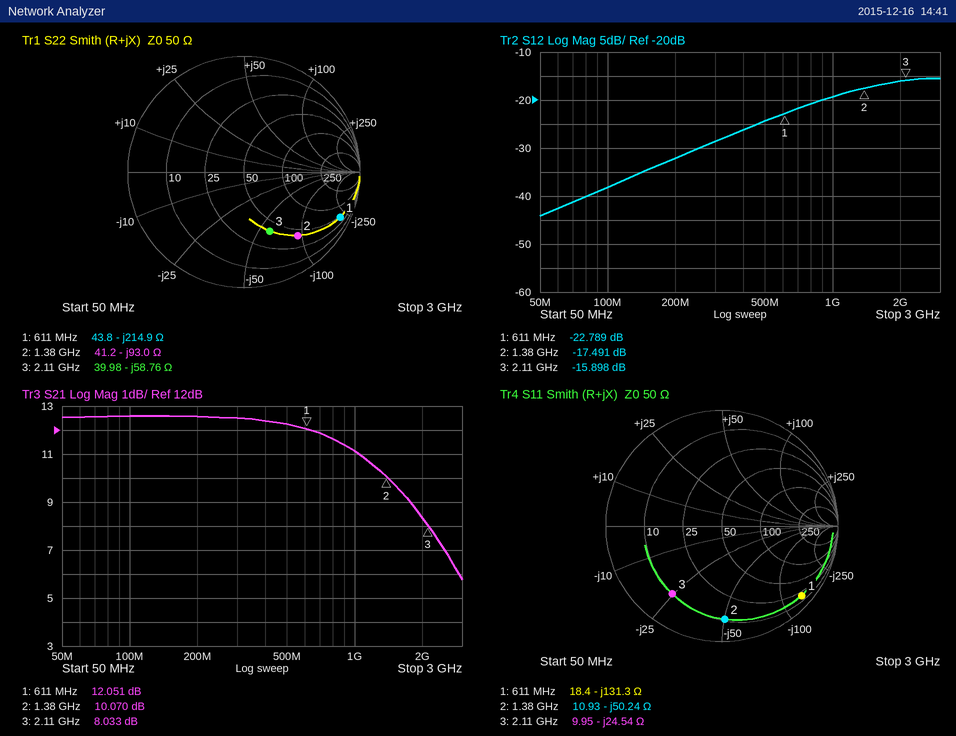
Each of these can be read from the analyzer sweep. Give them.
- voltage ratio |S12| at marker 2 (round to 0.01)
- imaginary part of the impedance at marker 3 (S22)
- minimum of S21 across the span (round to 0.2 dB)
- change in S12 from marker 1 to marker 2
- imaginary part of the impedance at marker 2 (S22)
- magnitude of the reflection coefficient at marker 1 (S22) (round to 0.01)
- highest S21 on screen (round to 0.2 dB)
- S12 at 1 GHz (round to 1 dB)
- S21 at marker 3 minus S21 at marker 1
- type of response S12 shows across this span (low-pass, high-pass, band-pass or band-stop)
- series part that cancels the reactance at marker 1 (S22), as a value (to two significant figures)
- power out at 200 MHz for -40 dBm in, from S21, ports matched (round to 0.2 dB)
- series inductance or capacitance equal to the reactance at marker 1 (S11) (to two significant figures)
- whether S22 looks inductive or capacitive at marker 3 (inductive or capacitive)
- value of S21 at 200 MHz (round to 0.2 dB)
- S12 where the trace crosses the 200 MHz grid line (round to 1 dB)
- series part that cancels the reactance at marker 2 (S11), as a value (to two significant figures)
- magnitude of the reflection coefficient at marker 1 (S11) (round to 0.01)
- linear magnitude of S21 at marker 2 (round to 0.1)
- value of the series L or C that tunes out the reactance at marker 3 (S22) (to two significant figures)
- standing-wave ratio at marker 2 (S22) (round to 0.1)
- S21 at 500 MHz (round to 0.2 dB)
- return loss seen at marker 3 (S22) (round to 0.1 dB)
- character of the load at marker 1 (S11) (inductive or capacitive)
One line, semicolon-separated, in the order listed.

0.13; -58.76 Ω; 5.8 dB; 5.298 dB; -93.0 Ω; 0.92; 12.6 dB; -19 dB; -4.018 dB; high-pass; 56 nH; -27.4 dBm; 2.0 pF; capacitive; 12.6 dB; -32 dB; 5.8 nH; 0.91; 3.2; 4.4 nH; 6.1; 12.2 dB; 5.1 dB; capacitive
